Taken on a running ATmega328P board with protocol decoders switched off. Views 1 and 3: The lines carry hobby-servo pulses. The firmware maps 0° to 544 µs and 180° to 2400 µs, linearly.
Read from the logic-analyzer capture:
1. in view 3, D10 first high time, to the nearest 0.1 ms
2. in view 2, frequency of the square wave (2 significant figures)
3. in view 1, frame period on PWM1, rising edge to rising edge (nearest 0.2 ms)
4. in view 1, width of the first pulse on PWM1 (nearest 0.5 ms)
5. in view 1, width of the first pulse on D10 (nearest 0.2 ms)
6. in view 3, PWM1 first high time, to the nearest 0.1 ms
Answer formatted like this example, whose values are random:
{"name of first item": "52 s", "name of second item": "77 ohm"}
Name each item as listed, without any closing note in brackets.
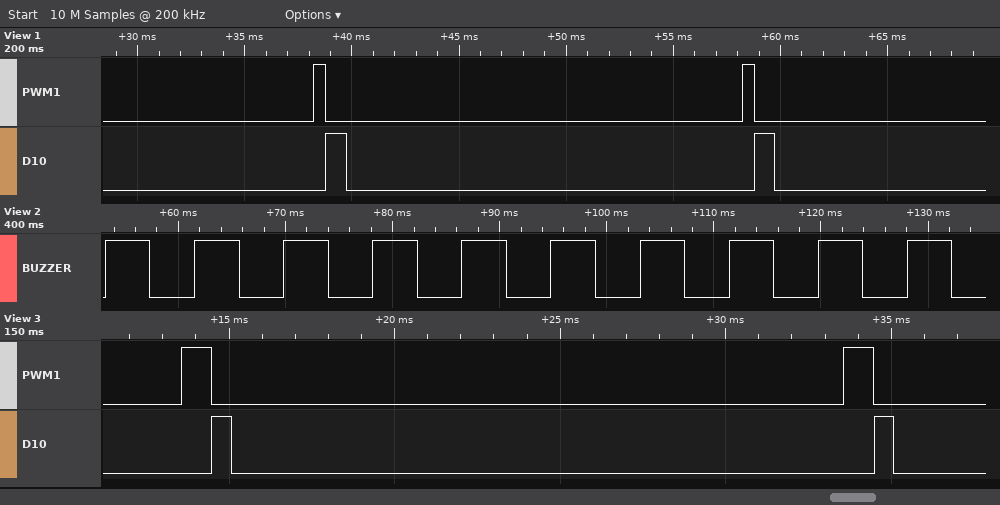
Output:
{"in view 3, D10 first high time, to the nearest 0.1 ms": "0.6 ms", "in view 2, frequency of the square wave": "120 Hz", "in view 1, frame period on PWM1, rising edge to rising edge": "20.0 ms", "in view 1, width of the first pulse on PWM1": "0.5 ms", "in view 1, width of the first pulse on D10": "1.0 ms", "in view 3, PWM1 first high time, to the nearest 0.1 ms": "0.9 ms"}
